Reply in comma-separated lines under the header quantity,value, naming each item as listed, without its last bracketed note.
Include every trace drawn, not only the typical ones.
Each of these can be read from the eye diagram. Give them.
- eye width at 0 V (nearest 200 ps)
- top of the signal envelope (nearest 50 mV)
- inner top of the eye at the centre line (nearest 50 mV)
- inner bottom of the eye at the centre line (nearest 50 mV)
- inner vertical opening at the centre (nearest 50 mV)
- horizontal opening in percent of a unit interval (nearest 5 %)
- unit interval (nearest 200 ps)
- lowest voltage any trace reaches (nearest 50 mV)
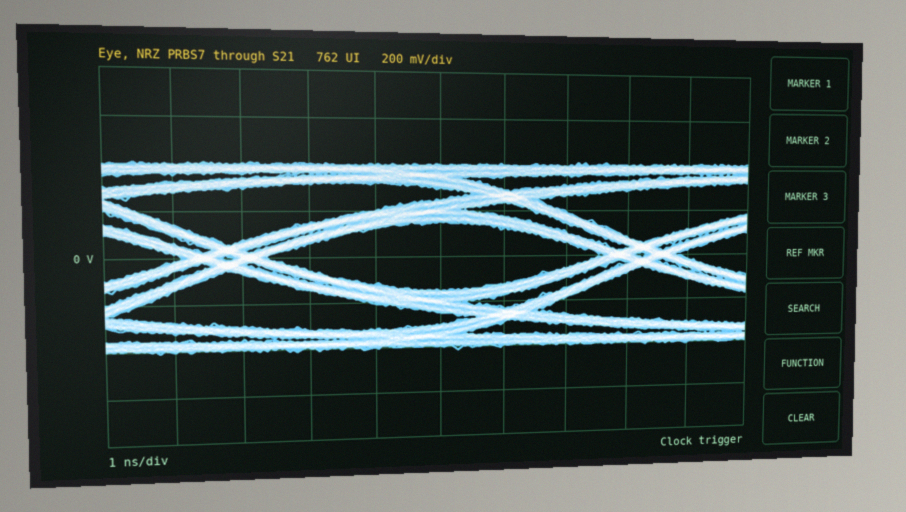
quantity,value
eye width at 0 V,5.2 ns
top of the signal envelope,400 mV
inner top of the eye at the centre line,150 mV
inner bottom of the eye at the centre line,-150 mV
inner vertical opening at the centre,300 mV
horizontal opening in percent of a unit interval,80 %
unit interval,6.4 ns
lowest voltage any trace reaches,-400 mV
